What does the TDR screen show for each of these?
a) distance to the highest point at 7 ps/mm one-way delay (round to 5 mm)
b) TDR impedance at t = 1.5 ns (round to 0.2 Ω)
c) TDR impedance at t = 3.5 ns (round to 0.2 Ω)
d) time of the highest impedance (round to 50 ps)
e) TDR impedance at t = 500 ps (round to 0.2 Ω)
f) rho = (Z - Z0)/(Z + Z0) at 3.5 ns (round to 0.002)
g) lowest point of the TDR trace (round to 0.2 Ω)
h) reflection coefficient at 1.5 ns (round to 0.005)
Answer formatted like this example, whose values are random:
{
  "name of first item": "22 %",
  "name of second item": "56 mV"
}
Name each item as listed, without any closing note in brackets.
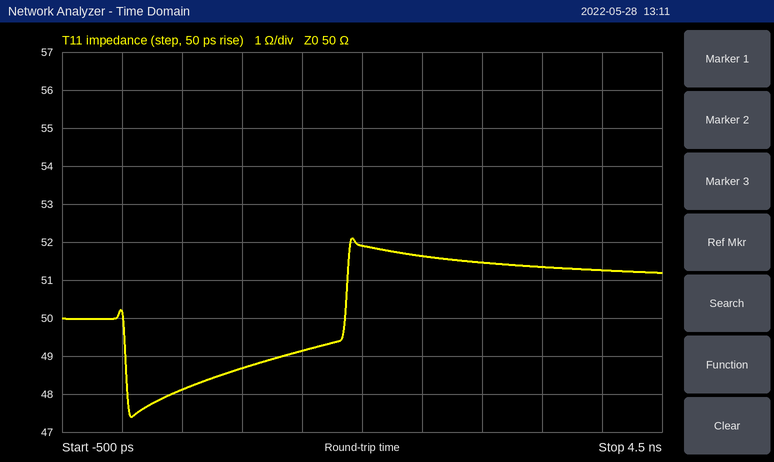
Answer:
{
  "distance to the highest point at 7 ps/mm one-way delay": "135 mm",
  "TDR impedance at t = 1.5 ns": "49.2 Ω",
  "TDR impedance at t = 3.5 ns": "51.4 Ω",
  "time of the highest impedance": "1.90 ns",
  "TDR impedance at t = 500 ps": "48.2 Ω",
  "rho = (Z - Z0)/(Z + Z0) at 3.5 ns": "+0.014",
  "lowest point of the TDR trace": "47.4 Ω",
  "reflection coefficient at 1.5 ns": "-0.010"
}
